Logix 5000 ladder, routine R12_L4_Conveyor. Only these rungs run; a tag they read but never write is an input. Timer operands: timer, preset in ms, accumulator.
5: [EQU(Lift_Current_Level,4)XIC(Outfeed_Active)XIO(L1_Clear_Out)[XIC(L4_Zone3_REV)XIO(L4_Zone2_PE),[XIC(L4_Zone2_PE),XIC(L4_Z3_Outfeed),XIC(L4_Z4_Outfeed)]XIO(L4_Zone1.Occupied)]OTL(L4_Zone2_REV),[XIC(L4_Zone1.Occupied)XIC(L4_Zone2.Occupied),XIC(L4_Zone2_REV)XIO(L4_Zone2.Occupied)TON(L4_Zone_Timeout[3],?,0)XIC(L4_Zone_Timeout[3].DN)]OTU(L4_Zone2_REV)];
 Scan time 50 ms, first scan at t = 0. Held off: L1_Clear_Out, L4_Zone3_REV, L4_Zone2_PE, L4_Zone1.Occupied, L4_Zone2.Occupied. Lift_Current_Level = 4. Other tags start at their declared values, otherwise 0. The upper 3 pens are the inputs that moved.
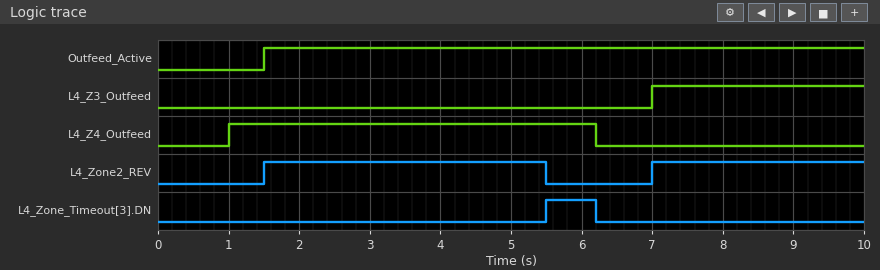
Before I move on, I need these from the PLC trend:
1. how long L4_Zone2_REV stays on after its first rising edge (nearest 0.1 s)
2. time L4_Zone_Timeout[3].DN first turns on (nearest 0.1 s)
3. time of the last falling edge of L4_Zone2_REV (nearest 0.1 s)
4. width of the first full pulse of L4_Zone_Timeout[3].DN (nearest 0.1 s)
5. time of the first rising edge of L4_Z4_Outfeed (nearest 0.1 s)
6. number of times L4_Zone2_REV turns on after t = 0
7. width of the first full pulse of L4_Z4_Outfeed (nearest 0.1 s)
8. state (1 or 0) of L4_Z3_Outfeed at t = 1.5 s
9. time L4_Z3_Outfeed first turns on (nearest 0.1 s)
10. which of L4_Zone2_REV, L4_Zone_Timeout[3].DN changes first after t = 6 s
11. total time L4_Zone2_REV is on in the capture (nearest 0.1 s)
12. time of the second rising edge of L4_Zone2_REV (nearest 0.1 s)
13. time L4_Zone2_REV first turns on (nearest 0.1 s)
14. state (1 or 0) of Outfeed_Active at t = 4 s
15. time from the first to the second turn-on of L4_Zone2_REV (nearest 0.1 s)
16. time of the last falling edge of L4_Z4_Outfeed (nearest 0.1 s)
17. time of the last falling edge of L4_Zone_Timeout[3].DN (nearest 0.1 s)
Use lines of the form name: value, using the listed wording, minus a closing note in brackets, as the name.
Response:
how long L4_Zone2_REV stays on after its first rising edge: 4.0 s
time L4_Zone_Timeout[3].DN first turns on: 5.5 s
time of the last falling edge of L4_Zone2_REV: 5.5 s
width of the first full pulse of L4_Zone_Timeout[3].DN: 0.7 s
time of the first rising edge of L4_Z4_Outfeed: 1.0 s
number of times L4_Zone2_REV turns on after t = 0: 2
width of the first full pulse of L4_Z4_Outfeed: 5.2 s
state (1 or 0) of L4_Z3_Outfeed at t = 1.5 s: 0
time L4_Z3_Outfeed first turns on: 7.0 s
which of L4_Zone2_REV, L4_Zone_Timeout[3].DN changes first after t = 6 s: L4_Zone_Timeout[3].DN
total time L4_Zone2_REV is on in the capture: 7.0 s
time of the second rising edge of L4_Zone2_REV: 7.0 s
time L4_Zone2_REV first turns on: 1.5 s
state (1 or 0) of Outfeed_Active at t = 4 s: 1
time from the first to the second turn-on of L4_Zone2_REV: 5.5 s
time of the last falling edge of L4_Z4_Outfeed: 6.2 s
time of the last falling edge of L4_Zone_Timeout[3].DN: 6.2 s
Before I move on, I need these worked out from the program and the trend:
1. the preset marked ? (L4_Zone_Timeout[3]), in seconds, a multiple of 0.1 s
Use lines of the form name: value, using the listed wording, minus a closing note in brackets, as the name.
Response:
the preset marked ? (L4_Zone_Timeout[3]), in seconds, a multiple of 0.1 s: 4.0 s
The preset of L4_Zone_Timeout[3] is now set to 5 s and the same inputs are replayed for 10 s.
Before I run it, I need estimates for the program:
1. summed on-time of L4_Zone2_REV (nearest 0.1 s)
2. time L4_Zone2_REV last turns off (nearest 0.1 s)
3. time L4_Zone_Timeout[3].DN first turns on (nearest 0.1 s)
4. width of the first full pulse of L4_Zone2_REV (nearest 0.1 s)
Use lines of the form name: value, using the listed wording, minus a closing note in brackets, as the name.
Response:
summed on-time of L4_Zone2_REV: 8.0 s
time L4_Zone2_REV last turns off: 6.5 s
time L4_Zone_Timeout[3].DN first turns on: 6.5 s
width of the first full pulse of L4_Zone2_REV: 5.0 s
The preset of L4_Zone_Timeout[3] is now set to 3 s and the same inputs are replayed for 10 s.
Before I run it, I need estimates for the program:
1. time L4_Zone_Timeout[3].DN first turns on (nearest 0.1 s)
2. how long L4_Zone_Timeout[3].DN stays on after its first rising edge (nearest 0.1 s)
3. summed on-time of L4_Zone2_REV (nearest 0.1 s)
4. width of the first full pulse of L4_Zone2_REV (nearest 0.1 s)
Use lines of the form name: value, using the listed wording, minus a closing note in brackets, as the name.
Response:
time L4_Zone_Timeout[3].DN first turns on: 4.5 s
how long L4_Zone_Timeout[3].DN stays on after its first rising edge: 1.7 s
summed on-time of L4_Zone2_REV: 6.0 s
width of the first full pulse of L4_Zone2_REV: 3.0 s
